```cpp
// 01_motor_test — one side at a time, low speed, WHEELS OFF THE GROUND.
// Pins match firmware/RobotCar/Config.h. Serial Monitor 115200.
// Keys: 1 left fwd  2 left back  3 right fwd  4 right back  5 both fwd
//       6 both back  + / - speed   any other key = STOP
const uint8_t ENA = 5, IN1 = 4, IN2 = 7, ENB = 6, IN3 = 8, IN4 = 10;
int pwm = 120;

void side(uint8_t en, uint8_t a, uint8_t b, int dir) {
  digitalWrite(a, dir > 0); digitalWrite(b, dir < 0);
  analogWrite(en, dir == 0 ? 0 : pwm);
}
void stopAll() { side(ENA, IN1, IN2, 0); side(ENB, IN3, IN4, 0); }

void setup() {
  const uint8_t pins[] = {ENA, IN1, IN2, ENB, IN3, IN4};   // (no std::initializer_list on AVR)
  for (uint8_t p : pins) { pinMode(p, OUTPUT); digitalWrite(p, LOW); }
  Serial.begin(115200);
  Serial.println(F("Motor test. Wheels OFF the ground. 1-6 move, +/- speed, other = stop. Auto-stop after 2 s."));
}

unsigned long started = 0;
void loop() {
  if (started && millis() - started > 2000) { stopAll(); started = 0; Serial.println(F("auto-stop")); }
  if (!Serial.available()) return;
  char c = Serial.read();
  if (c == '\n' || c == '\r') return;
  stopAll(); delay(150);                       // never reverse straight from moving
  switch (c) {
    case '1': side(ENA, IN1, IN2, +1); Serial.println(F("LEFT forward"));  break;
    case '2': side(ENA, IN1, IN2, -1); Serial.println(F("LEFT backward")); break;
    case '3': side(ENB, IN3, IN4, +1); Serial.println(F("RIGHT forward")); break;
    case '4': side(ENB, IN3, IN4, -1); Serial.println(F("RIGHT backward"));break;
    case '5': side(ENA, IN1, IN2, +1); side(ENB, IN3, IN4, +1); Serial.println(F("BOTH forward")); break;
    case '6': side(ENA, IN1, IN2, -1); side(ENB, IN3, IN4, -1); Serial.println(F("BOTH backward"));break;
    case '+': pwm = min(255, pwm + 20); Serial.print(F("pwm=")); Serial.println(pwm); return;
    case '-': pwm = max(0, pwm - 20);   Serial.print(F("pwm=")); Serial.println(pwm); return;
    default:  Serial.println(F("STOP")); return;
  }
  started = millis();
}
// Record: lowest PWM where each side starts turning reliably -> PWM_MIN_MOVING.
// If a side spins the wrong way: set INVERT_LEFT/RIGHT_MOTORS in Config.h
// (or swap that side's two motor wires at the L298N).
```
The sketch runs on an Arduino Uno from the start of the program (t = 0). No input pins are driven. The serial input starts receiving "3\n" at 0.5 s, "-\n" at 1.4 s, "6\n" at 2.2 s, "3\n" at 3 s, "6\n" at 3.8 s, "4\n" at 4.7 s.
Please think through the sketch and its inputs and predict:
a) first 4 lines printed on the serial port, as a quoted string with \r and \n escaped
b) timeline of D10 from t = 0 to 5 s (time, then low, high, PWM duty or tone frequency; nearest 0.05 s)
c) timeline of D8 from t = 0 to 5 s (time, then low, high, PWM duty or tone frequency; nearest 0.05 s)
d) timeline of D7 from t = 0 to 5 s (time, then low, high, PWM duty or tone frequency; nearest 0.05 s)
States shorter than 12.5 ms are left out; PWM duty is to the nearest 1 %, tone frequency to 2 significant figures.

"Motor test. Wheels OFF the ground. 1-6 move, +/- speed, other = stop. Auto-stop after 2 s.\r\nRIGHT forward\r\npwm=100\r\nBOTH backward\r\n"
0 s low; 2.35 s high; 3 s low; 3.95 s high; 4.7 s low; 4.85 s high
0 s low; 0.65 s high; 1.4 s low; 3.15 s high; 3.8 s low
0 s low; 2.35 s high; 3 s low; 3.95 s high; 4.7 s low
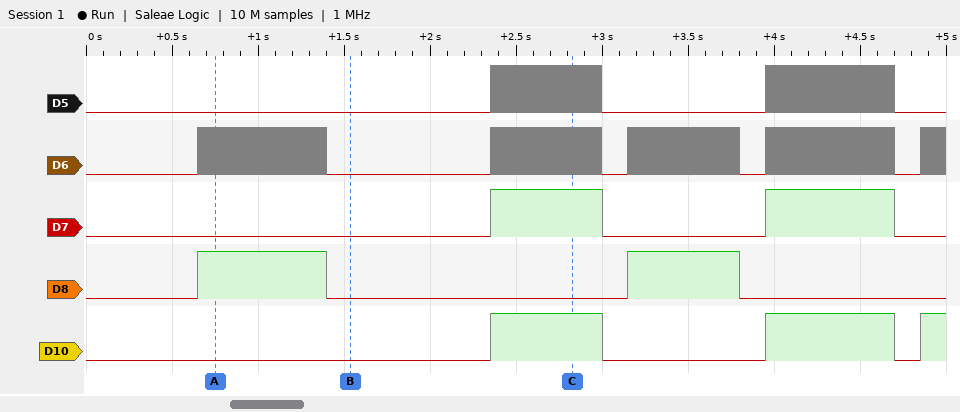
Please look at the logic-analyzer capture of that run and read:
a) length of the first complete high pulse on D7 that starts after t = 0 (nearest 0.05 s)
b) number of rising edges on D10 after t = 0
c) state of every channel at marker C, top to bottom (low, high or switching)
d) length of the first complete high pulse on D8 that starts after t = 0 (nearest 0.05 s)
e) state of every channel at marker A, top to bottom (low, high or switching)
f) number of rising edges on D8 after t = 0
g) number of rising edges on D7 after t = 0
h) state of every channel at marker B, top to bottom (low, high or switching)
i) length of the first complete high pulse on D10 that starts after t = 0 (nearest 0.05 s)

0.65 s
3
D5 switching, D6 switching, D7 high, D8 low, D10 high
0.75 s
D5 low, D6 switching, D7 low, D8 high, D10 low
2
2
D5 low, D6 low, D7 low, D8 low, D10 low
0.65 s
